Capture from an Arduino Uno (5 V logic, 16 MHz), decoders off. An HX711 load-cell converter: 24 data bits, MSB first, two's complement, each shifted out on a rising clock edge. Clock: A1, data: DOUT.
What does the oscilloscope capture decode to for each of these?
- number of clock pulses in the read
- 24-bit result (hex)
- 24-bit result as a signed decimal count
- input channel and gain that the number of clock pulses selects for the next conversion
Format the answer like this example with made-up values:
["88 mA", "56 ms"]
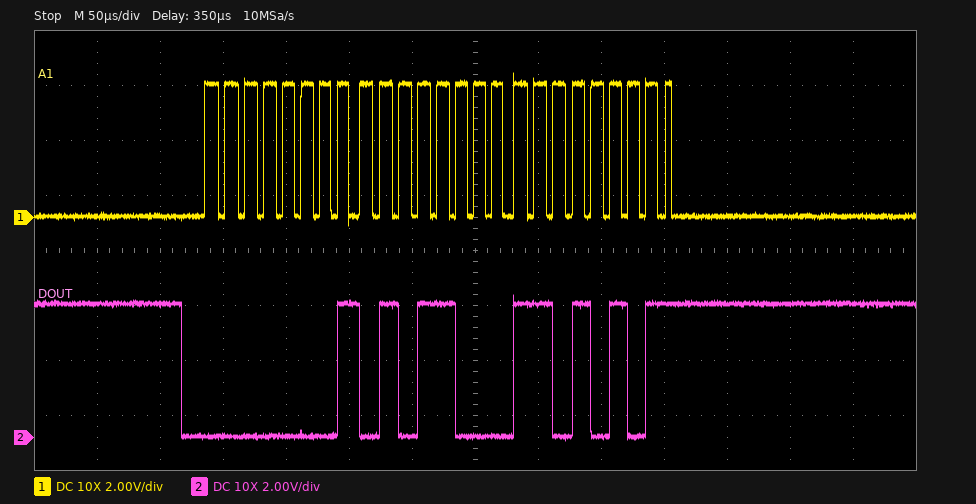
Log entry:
["25", "0x0158D5", "88277", "channel A, gain 128"]
